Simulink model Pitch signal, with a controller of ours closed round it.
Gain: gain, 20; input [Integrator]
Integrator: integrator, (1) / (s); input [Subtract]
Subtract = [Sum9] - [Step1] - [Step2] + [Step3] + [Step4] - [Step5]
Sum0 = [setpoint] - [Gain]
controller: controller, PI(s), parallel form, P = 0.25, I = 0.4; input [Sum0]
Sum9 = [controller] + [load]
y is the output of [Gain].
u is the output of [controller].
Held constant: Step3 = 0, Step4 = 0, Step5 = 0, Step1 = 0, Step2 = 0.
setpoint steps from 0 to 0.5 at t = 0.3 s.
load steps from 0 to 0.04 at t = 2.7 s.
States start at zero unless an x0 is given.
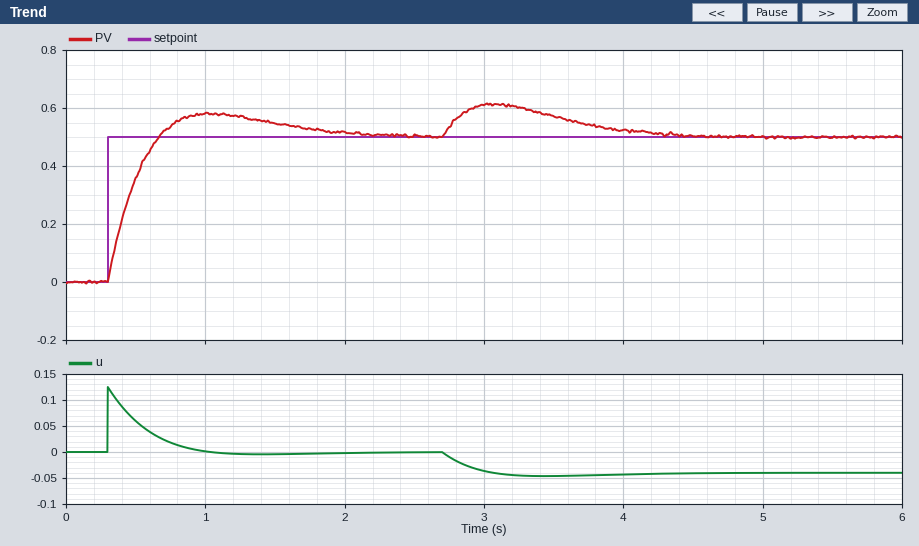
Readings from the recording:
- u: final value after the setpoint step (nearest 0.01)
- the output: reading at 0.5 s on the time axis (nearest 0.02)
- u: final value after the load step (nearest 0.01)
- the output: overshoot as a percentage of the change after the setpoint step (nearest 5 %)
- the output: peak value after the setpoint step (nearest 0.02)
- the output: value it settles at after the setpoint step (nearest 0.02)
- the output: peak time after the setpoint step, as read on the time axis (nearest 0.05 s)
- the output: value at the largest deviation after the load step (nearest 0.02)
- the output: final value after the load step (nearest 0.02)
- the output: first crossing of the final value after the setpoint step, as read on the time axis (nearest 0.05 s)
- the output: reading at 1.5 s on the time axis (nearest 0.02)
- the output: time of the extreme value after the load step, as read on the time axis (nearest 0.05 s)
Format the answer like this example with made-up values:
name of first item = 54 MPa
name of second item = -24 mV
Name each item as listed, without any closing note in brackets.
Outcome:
u: final value after the setpoint step = 0.00
the output: reading at 0.5 s on the time axis = 0.36
u: final value after the load step = -0.04
the output: overshoot as a percentage of the change after the setpoint step = 15 %
the output: peak value after the setpoint step = 0.58
the output: value it settles at after the setpoint step = 0.50
the output: peak time after the setpoint step, as read on the time axis = 1.05 s
the output: value at the largest deviation after the load step = 0.62
the output: final value after the load step = 0.50
the output: first crossing of the final value after the setpoint step, as read on the time axis = 0.65 s
the output: reading at 1.5 s on the time axis = 0.54
the output: time of the extreme value after the load step, as read on the time axis = 3.05 s
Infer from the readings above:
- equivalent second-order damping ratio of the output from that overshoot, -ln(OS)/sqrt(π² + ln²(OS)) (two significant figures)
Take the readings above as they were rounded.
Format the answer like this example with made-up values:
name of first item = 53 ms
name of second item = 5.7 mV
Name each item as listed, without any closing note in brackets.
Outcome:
equivalent second-order damping ratio of the output from that overshoot, -ln(OS)/sqrt(π² + ln²(OS)) = 0.52
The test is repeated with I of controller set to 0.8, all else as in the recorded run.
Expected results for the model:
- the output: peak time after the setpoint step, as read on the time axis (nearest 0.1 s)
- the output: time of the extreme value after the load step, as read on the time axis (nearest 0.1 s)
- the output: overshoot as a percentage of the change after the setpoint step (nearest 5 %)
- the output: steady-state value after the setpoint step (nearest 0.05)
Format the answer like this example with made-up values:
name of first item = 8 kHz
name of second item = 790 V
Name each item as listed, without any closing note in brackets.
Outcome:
the output: peak time after the setpoint step, as read on the time axis = 0.9 s
the output: time of the extreme value after the load step, as read on the time axis = 3.0 s
the output: overshoot as a percentage of the change after the setpoint step = 25 %
the output: steady-state value after the setpoint step = 0.50
